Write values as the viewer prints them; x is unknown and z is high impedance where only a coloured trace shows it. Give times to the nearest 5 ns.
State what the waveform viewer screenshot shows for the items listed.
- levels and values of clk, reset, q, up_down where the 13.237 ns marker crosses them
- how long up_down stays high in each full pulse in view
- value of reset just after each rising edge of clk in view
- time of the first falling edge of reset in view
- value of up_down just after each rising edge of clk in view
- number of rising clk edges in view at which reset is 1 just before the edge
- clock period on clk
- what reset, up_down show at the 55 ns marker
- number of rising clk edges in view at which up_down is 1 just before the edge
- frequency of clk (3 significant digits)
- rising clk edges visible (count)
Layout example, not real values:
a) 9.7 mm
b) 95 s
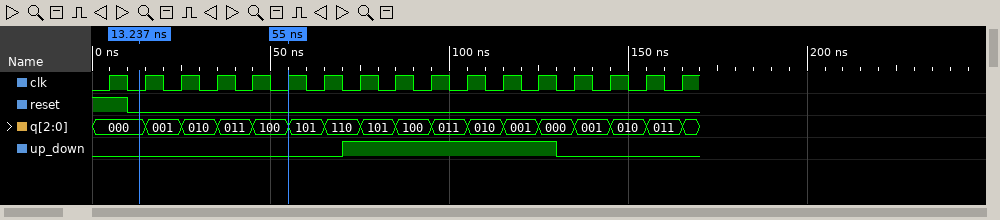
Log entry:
a) clk=0, reset=0, q=000, up_down=0
b) 60 ns
c) 1 0 0 0 0 0 0 0 0 0 0 0 0 0 0 0 0
d) 10 ns
e) 0 0 0 0 0 0 0 1 1 1 1 1 1 0 0 0 0
f) 1
g) 10 ns
h) reset=0, up_down=0
i) 6
j) 100 MHz
k) 17
